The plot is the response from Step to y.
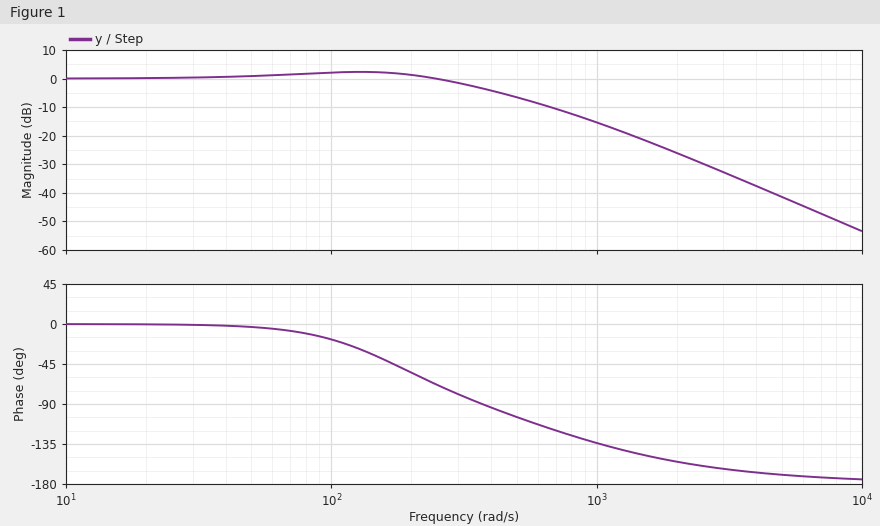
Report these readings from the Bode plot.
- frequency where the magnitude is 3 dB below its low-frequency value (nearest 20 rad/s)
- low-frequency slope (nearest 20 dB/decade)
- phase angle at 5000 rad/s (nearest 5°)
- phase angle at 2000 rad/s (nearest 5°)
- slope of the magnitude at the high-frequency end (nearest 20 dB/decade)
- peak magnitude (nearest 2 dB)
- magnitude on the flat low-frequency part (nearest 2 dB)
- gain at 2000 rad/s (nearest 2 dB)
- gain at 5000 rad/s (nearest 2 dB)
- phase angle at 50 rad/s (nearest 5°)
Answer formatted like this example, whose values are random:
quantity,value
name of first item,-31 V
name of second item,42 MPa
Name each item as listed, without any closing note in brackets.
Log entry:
quantity,value
frequency where the magnitude is 3 dB below its low-frequency value,360 rad/s
low-frequency slope,0 dB/decade
phase angle at 5000 rad/s,-170°
phase angle at 2000 rad/s,-155°
slope of the magnitude at the high-frequency end,-40 dB/decade
peak magnitude,2 dB
magnitude on the flat low-frequency part,0 dB
gain at 2000 rad/s,-26 dB
gain at 5000 rad/s,-42 dB
phase angle at 50 rad/s,-5°
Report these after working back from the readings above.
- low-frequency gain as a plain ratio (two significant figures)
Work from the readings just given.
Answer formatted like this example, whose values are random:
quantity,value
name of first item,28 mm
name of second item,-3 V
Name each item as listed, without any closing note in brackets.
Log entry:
quantity,value
low-frequency gain as a plain ratio,1.0
